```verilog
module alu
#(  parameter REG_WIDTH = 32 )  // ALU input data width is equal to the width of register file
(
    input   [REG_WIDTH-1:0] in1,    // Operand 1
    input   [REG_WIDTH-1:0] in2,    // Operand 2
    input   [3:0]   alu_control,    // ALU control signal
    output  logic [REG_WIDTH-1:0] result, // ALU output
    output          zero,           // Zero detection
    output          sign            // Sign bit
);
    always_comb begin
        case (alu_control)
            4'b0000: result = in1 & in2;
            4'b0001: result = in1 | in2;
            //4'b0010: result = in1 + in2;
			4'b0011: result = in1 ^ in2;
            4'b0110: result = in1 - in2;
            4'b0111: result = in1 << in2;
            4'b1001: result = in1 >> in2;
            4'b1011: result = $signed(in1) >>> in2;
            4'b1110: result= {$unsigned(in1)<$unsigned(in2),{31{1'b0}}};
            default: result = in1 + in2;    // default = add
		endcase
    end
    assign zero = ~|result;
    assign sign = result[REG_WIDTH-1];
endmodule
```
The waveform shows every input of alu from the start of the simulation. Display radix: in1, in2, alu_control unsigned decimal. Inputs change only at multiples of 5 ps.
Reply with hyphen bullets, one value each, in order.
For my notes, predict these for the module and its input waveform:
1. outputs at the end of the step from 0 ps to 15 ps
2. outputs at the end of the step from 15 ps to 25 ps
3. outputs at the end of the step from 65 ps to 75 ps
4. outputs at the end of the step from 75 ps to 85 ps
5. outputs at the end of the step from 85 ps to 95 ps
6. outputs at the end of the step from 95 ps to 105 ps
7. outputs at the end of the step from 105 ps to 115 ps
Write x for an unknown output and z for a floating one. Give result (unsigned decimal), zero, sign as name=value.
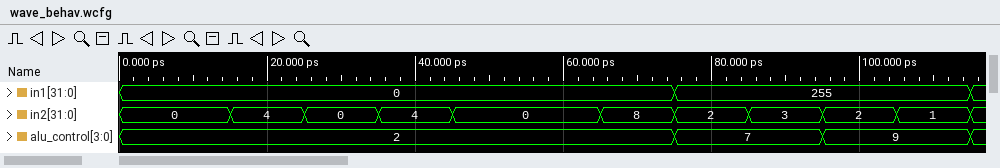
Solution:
- result=0, zero=1, sign=0
- result=4, zero=0, sign=0
- result=8, zero=0, sign=0
- result=1020, zero=0, sign=0
- result=2040, zero=0, sign=0
- result=63, zero=0, sign=0
- result=127, zero=0, sign=0
